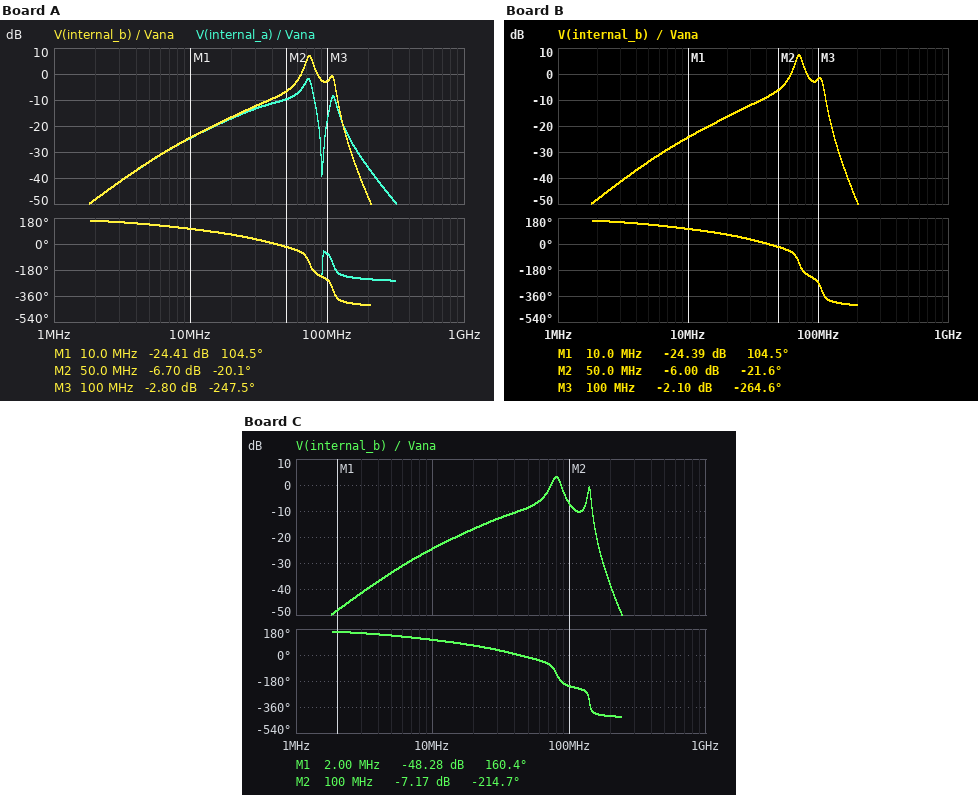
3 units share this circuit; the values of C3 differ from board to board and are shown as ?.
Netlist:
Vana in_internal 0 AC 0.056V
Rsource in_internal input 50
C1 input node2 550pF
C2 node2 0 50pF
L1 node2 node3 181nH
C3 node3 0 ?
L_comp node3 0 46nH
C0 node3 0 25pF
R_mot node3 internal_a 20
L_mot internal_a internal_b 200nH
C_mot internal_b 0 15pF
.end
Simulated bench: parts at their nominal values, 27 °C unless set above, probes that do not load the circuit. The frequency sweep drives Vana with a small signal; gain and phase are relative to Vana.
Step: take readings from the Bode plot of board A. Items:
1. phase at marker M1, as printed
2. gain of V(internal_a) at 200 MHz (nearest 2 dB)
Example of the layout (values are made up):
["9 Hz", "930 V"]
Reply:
["104.5 deg", "-36 dB"]
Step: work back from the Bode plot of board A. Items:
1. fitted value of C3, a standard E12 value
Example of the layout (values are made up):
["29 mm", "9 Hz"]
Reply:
["68 pF"]
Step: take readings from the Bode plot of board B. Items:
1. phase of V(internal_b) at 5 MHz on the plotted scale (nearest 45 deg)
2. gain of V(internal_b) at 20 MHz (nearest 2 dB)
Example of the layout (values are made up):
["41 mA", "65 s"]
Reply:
["135 deg", "-16 dB"]
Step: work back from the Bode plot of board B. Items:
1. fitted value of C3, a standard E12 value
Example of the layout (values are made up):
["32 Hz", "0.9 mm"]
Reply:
["82 pF"]
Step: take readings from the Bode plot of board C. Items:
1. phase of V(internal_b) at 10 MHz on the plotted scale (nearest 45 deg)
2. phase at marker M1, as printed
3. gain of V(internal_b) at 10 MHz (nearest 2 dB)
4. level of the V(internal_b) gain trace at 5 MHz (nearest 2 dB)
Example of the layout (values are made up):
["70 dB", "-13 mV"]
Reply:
["90 deg", "160.4 deg", "-24 dB", "-34 dB"]
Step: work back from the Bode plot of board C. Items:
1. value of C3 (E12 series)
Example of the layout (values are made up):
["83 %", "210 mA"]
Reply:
["22 pF"]
